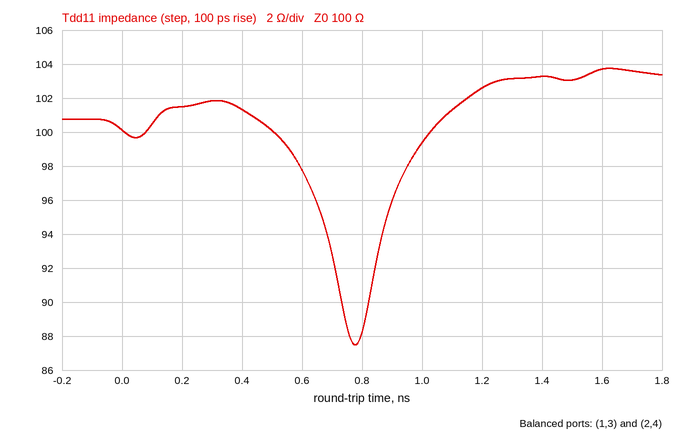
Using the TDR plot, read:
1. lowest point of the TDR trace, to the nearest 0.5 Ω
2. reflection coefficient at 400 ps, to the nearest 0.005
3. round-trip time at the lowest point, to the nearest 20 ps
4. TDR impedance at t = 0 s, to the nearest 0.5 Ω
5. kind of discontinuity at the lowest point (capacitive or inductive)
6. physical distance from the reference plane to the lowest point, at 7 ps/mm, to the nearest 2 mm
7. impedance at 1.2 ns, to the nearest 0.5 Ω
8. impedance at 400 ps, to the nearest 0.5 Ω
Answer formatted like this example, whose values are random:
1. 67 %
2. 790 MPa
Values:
1. 87.5 Ω
2. +0.005
3. 780 ps
4. 100.0 Ω
5. capacitive
6. 56 mm
7. 102.5 Ω
8. 101.5 Ω
